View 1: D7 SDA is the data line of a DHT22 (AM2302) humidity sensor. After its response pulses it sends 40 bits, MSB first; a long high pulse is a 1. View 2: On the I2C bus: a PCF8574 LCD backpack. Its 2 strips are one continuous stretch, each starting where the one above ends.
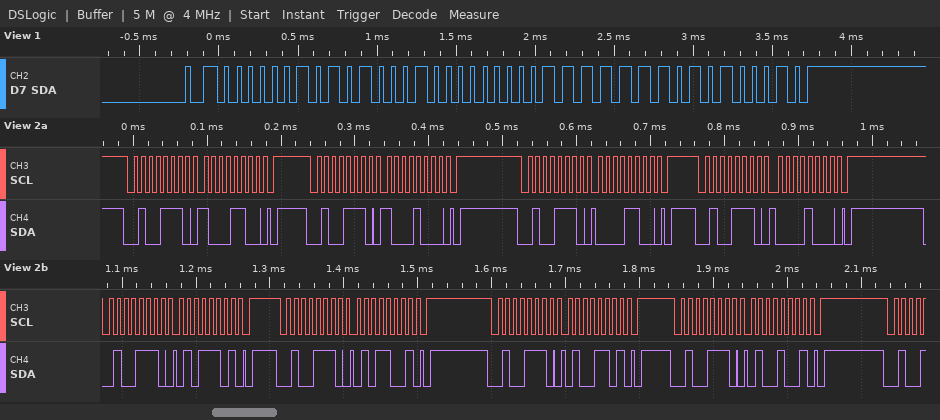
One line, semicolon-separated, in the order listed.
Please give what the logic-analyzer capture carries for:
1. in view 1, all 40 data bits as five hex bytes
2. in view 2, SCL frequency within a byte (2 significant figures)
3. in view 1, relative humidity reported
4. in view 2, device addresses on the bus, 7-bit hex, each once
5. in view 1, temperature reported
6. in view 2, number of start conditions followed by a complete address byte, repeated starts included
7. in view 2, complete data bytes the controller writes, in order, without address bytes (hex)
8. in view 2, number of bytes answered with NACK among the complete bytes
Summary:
02 A2 00 FE A2; 100 kHz; 67.4 %; 0x27; 25.4 °C; 8; 8C 88 0C 08 5D 59 4D 49; 0
